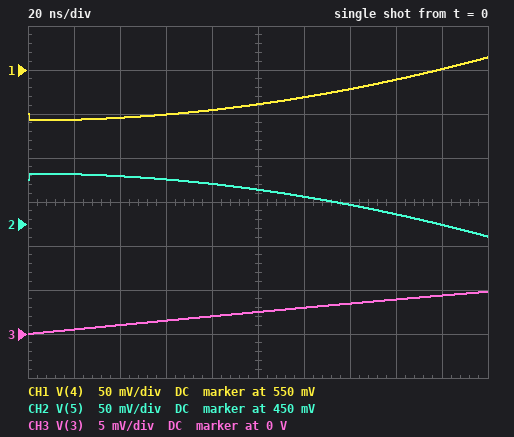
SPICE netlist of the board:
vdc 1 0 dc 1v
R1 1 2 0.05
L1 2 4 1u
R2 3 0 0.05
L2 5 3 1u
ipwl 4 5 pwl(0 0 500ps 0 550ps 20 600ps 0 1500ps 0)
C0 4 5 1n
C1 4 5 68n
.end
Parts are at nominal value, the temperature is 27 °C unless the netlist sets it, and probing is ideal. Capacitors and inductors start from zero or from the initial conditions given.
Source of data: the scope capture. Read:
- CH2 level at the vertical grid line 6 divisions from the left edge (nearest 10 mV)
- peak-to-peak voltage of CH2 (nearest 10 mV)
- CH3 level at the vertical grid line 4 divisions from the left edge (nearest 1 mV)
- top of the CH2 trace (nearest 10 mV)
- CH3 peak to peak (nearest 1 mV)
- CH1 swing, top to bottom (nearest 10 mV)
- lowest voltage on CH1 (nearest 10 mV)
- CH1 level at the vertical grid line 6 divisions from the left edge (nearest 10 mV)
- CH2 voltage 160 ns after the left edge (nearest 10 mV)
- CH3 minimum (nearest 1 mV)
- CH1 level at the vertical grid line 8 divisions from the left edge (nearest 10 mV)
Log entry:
480 mV
70 mV
2 mV
510 mV
5 mV
70 mV
490 mV
520 mV
460 mV
0 V
540 mV
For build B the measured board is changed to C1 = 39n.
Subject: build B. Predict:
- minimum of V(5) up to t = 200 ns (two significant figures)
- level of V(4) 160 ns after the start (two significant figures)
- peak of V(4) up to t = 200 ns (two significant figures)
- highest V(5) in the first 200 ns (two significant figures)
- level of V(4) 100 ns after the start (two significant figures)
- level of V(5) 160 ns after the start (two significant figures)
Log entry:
390 mV
570 mV
610 mV
510 mV
520 mV
430 mV
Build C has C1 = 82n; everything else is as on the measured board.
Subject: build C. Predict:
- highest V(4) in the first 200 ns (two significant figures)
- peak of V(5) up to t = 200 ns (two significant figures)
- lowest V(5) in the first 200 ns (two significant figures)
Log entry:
550 mV
510 mV
450 mV
